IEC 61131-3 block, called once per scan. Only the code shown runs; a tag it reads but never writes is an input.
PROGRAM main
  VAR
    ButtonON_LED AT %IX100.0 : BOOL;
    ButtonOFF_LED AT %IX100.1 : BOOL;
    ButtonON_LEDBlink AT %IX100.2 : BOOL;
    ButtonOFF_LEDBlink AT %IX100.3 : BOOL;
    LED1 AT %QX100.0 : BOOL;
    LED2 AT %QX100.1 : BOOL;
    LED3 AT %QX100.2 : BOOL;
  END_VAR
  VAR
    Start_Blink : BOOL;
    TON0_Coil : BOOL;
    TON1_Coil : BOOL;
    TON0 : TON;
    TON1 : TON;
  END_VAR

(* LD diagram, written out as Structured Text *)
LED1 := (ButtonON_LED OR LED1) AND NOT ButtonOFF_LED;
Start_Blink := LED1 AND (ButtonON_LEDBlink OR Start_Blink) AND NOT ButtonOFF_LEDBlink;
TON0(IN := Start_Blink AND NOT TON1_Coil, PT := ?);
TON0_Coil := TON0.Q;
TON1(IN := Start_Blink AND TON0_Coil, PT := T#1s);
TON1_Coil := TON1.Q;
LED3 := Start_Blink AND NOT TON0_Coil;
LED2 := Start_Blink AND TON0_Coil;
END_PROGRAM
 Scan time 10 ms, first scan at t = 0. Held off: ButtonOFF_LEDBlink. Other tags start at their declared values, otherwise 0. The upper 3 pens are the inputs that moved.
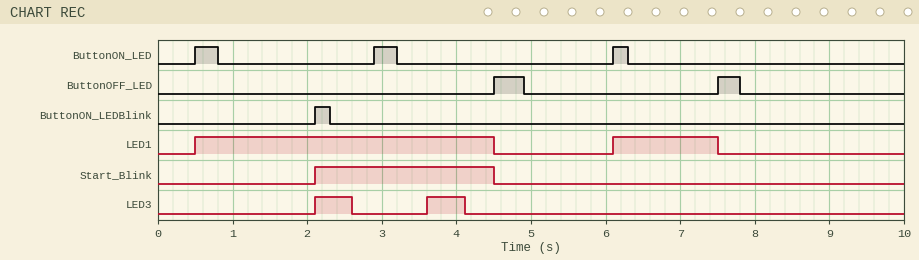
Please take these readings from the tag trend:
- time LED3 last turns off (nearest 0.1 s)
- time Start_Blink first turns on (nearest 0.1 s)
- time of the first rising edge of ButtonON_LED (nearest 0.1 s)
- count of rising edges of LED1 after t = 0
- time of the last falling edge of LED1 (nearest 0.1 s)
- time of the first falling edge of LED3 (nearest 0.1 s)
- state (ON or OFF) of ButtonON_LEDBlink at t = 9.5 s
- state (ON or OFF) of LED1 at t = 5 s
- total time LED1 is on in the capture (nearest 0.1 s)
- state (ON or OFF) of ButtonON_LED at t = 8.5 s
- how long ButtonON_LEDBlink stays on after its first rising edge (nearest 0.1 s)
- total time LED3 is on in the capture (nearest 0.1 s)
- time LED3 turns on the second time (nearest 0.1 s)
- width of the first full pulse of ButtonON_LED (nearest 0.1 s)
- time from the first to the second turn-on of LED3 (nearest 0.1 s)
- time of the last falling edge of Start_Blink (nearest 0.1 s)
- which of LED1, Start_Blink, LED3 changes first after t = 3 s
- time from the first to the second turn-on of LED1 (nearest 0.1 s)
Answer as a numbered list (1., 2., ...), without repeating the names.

1. 4.1 s
2. 2.1 s
3. 0.5 s
4. 2
5. 7.5 s
6. 2.6 s
7. OFF
8. OFF
9. 5.4 s
10. OFF
11. 0.2 s
12. 1.0 s
13. 3.6 s
14. 0.3 s
15. 1.5 s
16. 4.5 s
17. LED3
18. 5.6 s
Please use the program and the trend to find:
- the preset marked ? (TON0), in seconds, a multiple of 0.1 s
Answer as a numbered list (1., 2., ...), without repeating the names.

1. 0.5 s
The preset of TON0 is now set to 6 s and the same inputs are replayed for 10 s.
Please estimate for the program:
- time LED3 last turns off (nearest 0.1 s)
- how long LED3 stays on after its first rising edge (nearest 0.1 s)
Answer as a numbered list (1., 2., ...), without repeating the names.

1. 4.5 s
2. 2.4 s
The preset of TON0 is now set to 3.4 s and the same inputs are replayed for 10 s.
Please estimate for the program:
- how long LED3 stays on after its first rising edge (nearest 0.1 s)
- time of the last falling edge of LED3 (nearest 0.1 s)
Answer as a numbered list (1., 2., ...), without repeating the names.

1. 2.4 s
2. 4.5 s
